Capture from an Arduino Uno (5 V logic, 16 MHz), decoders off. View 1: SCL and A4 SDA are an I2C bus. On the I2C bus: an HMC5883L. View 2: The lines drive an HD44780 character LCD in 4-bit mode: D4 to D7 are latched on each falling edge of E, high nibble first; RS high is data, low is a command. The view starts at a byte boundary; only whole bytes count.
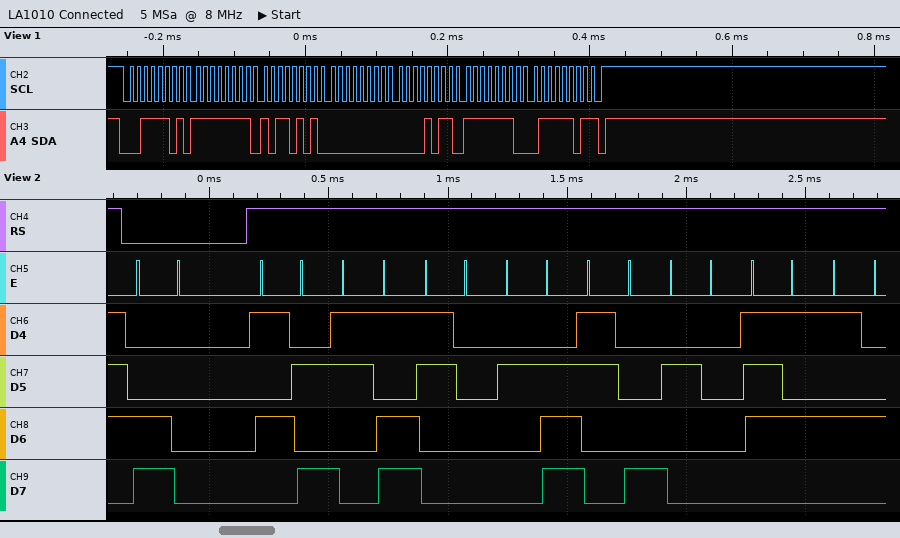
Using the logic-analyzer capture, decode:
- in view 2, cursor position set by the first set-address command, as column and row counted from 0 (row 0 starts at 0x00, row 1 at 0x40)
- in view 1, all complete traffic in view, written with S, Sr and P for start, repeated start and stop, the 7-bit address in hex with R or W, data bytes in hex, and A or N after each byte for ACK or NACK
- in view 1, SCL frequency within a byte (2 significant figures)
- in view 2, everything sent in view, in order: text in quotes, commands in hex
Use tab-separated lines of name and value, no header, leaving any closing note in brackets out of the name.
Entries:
in view 2, cursor position set by the first set-address command, as column and row counted from 0	column 0, row 1
in view 1, all complete traffic in view, written with S, Sr and P for start, repeated start and stop, the 7-bit address in hex with R or W, data bytes in hex, and A or N after each byte for ACK or NACK	S 1ER A FF A B5 A 00 A 0B A FE A 7D N P
in view 1, SCL frequency within a byte	100 kHz
in view 2, everything sent in view, in order: text in quotes, commands in hex	0xC0 "Z=0.8 uT"
